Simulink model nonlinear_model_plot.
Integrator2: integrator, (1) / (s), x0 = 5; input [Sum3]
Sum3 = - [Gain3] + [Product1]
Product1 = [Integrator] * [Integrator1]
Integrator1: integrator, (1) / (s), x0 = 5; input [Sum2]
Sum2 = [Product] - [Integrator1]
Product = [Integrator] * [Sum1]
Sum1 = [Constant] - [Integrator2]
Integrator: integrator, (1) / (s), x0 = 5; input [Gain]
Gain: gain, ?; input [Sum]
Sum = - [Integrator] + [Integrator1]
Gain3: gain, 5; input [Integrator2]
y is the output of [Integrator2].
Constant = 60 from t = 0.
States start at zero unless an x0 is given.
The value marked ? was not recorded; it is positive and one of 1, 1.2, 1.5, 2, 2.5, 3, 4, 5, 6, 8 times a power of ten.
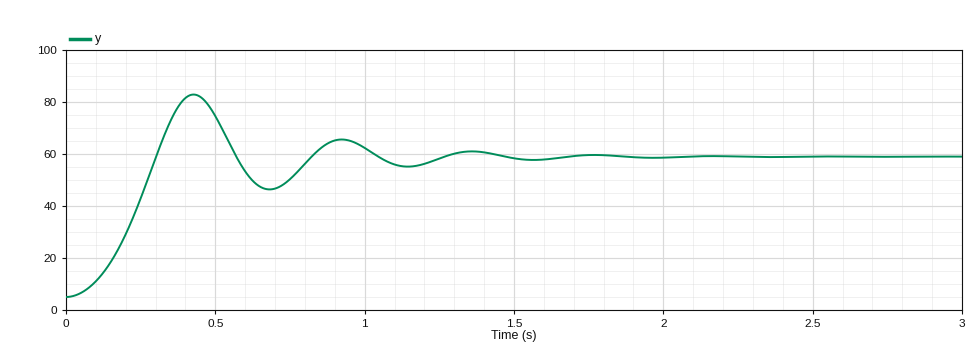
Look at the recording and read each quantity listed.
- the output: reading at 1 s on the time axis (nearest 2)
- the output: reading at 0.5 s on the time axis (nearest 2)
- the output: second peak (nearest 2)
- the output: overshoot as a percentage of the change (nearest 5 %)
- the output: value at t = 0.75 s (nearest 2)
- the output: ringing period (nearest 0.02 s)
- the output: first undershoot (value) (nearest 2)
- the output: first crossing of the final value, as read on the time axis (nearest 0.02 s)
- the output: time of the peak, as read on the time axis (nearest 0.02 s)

62
74
66
45 %
50
0.50 s
46
0.30 s
0.42 s
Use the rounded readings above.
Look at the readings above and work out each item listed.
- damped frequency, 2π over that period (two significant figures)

13 rad/s
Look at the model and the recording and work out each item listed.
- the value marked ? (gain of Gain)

0.5
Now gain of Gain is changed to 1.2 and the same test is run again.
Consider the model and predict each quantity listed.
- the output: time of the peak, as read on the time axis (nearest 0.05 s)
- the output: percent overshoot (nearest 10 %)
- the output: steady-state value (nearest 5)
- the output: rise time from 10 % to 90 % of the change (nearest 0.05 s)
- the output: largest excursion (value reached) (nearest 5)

0.35 s
60 %
60
0.15 s
90
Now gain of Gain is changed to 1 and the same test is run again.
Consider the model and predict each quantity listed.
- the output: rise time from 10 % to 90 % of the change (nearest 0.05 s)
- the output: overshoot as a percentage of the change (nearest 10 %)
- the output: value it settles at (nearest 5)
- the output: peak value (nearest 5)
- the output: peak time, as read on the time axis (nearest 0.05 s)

0.15 s
60 %
60
90
0.35 s
